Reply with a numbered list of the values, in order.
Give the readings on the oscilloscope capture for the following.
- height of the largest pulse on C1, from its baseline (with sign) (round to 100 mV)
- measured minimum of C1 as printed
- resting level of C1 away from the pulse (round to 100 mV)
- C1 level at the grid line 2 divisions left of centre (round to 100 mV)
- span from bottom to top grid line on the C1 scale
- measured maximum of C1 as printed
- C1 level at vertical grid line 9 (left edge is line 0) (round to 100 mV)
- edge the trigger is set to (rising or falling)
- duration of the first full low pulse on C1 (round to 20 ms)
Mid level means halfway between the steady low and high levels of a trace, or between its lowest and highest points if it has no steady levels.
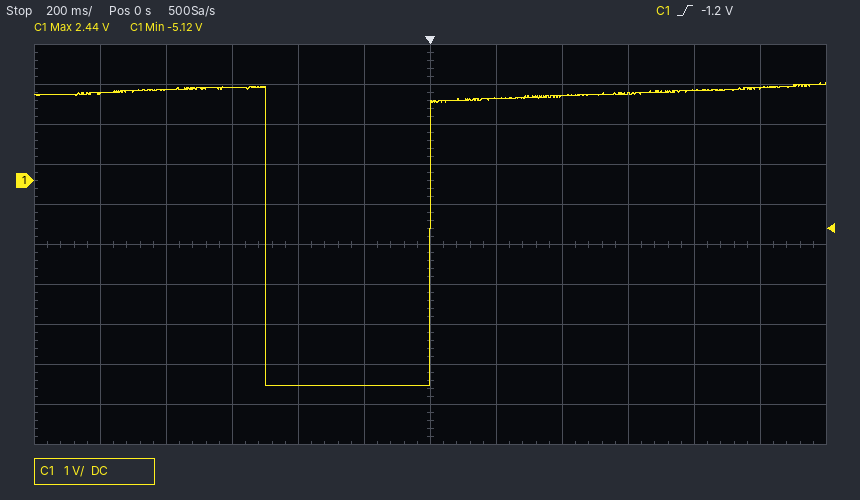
1. -7.3 V
2. -5.12 V
3. 2.2 V
4. -5.1 V
5. 10 V
6. 2.44 V
7. 2.2 V
8. rising
9. 500 ms
